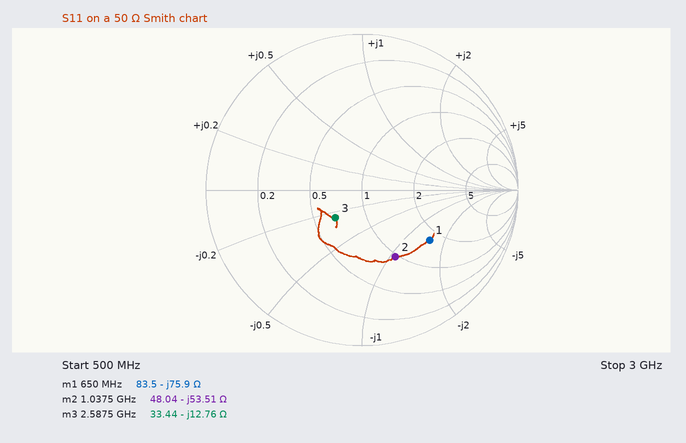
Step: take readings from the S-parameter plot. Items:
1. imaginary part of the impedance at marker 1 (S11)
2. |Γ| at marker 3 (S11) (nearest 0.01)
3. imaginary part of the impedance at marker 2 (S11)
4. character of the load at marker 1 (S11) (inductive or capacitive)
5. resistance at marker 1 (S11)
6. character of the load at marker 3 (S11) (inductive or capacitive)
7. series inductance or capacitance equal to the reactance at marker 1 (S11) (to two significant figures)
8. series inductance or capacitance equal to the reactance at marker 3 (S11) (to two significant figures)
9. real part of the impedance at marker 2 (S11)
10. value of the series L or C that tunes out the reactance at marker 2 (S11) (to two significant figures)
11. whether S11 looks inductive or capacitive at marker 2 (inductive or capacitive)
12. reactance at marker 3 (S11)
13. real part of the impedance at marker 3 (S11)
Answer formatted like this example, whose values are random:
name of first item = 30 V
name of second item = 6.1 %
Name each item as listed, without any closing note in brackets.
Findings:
imaginary part of the impedance at marker 1 = -75.9 Ω
|Γ| at marker 3 (S11) = 0.25
imaginary part of the impedance at marker 2 = -53.51 Ω
character of the load at marker 1 (S11) = capacitive
resistance at marker 1 = 83.5 Ω
character of the load at marker 3 (S11) = capacitive
series inductance or capacitance equal to the reactance at marker 1 (S11) = 3.2 pF
series inductance or capacitance equal to the reactance at marker 3 (S11) = 4.8 pF
real part of the impedance at marker 2 = 48.04 Ω
value of the series L or C that tunes out the reactance at marker 2 (S11) = 8.2 nH
whether S11 looks inductive or capacitive at marker 2 = capacitive
reactance at marker 3 = -12.76 Ω
real part of the impedance at marker 3 = 33.44 Ω
